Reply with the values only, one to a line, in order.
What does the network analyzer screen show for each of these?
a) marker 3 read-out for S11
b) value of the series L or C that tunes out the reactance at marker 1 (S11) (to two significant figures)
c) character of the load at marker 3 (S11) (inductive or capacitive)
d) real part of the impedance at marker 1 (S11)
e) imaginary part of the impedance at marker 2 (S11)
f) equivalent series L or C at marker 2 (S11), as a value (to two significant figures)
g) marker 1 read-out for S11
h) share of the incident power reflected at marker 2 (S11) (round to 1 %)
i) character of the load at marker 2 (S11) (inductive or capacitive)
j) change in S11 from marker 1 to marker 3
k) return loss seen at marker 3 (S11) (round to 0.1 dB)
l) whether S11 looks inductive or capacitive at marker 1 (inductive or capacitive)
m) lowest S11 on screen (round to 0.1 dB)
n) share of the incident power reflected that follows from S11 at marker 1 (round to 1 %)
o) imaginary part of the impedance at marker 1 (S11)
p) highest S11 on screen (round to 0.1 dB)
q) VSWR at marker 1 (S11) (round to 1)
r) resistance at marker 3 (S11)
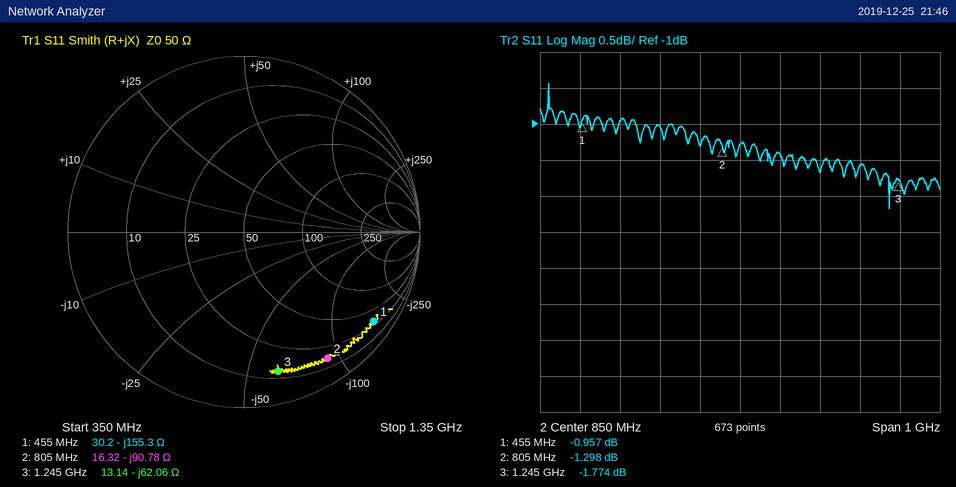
-1.774 dB
54 nH
capacitive
30.2 Ω
-90.78 Ω
2.2 pF
-0.957 dB
74 %
capacitive
-0.817 dB
1.8 dB
capacitive
-2.2 dB
80 %
-155.3 Ω
-0.4 dB
18
13.14 Ω
